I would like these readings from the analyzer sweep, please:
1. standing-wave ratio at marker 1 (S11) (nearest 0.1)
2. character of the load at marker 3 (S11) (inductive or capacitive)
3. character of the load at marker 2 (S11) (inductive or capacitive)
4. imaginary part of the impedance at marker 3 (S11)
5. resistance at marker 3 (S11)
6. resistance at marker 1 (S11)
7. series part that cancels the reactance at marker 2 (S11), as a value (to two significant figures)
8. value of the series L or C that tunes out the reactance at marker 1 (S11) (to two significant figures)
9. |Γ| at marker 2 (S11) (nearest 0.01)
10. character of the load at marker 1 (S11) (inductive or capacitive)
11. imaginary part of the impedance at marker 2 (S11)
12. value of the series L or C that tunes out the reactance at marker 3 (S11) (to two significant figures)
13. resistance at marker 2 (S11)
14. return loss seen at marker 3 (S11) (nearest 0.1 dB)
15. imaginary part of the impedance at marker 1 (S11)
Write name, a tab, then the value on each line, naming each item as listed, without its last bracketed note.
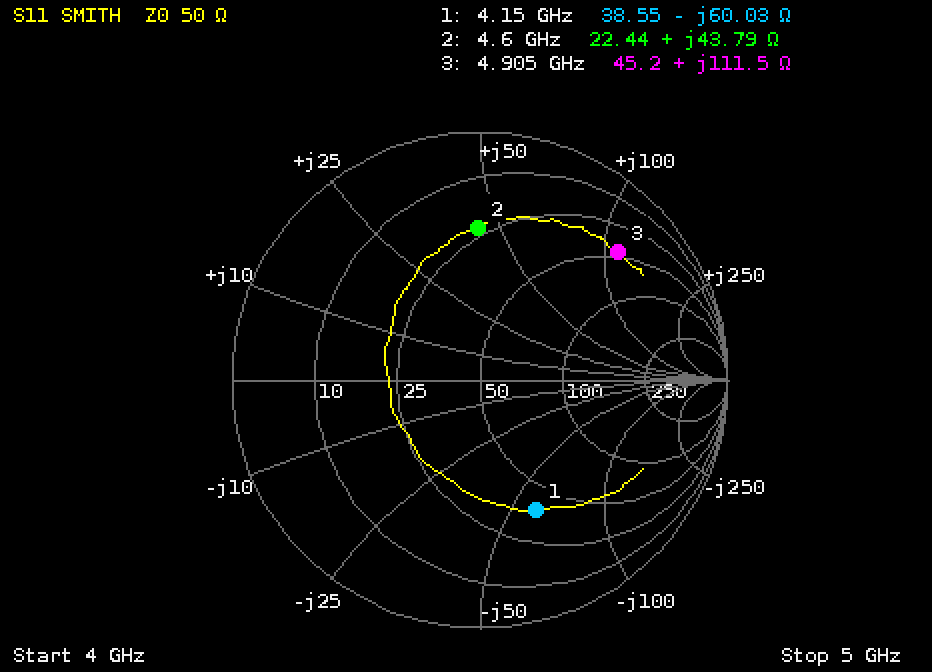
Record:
standing-wave ratio at marker 1 (S11)	3.7
character of the load at marker 3 (S11)	inductive
character of the load at marker 2 (S11)	inductive
imaginary part of the impedance at marker 3	+111.5 Ω
resistance at marker 3	45.2 Ω
resistance at marker 1	38.55 Ω
series part that cancels the reactance at marker 2 (S11), as a value	790 fF
value of the series L or C that tunes out the reactance at marker 1 (S11)	2.3 nH
|Γ| at marker 2 (S11)	0.61
character of the load at marker 1 (S11)	capacitive
imaginary part of the impedance at marker 2	+43.79 Ω
value of the series L or C that tunes out the reactance at marker 3 (S11)	290 fF
resistance at marker 2	22.44 Ω
return loss seen at marker 3 (S11)	2.4 dB
imaginary part of the impedance at marker 1	-60.03 Ω
